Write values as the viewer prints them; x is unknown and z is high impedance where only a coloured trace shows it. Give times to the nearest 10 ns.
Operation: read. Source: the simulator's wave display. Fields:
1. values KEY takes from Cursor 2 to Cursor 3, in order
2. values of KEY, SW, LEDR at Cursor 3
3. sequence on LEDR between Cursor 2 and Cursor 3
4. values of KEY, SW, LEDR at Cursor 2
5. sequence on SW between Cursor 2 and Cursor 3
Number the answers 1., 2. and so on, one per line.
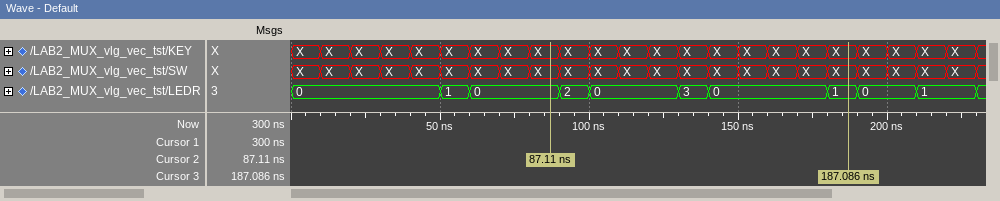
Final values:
1. X, X, X, X, X, X, X, X, X, X, X
2. KEY=X, SW=X, LEDR=1
3. 0, 2, 0, 3, 0, 1
4. KEY=X, SW=X, LEDR=0
5. X, X, X, X, X, X, X, X, X, X, X
